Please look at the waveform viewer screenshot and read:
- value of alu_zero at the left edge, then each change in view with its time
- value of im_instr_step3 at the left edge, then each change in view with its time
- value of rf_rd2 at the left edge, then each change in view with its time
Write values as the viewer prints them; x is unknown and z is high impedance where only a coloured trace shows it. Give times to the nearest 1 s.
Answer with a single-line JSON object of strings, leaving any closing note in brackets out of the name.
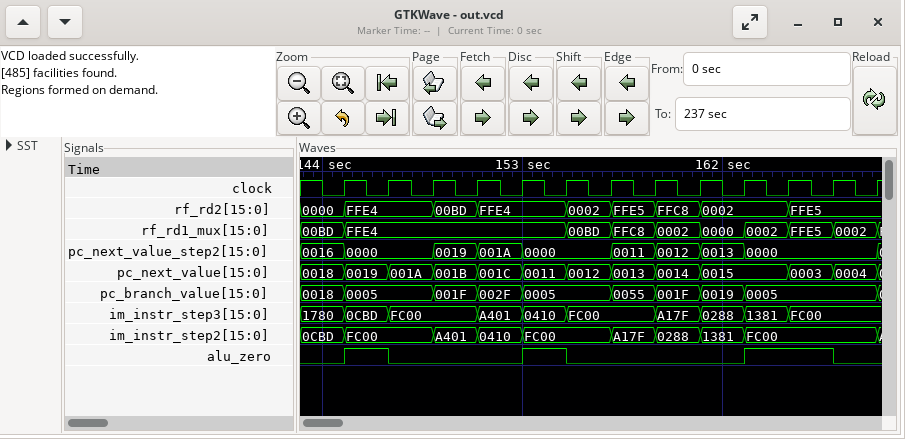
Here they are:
{"value of alu_zero at the left edge, then each change in view with its time": "0, 1 at 145 s, 0 at 147 s, 1 at 153 s, 0 at 155 s, 1 at 163 s, 0 at 167 s", "value of im_instr_step3 at the left edge, then each change in view with its time": "1780, 0CBD at 145 s, FC00 at 147 s, A401 at 151 s, 0410 at 153 s, FC00 at 155 s, A17F at 159 s, 0288 at 161 s, 1381 at 163 s, FC00 at 165 s", "value of rf_rd2 at the left edge, then each change in view with its time": "0000, FFE4 at 145 s, 00BD at 149 s, FFE4 at 151 s, 0002 at 155 s, FFE5 at 157 s, FFC8 at 159 s, 0002 at 161 s, FFE5 at 165 s"}
